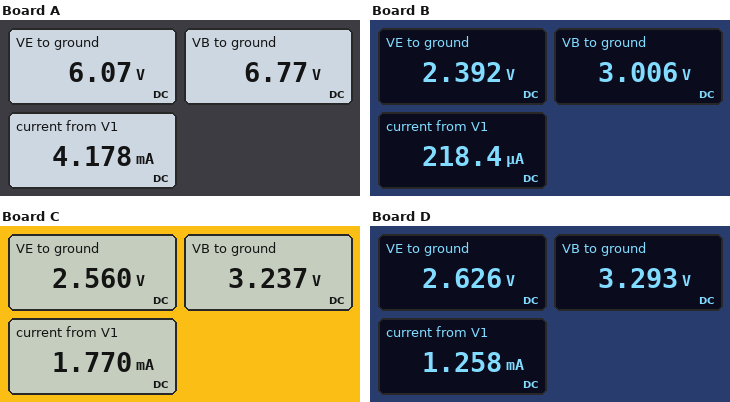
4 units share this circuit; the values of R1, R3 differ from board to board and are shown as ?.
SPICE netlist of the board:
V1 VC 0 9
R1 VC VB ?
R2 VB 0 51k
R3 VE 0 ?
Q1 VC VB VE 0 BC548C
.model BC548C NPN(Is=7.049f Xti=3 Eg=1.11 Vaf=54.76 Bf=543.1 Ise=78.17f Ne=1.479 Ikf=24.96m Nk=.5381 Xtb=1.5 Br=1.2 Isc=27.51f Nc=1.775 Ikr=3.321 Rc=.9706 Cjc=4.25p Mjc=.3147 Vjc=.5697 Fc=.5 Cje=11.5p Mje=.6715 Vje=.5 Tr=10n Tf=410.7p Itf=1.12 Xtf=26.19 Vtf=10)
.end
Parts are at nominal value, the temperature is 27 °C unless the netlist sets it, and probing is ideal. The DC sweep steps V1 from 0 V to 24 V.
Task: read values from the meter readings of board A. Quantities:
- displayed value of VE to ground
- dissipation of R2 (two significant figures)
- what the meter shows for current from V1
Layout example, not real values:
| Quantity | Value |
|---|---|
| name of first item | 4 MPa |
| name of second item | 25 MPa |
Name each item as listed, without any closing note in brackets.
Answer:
| Quantity | Value |
|---|---|
| displayed value of VE to ground | 6.07 V |
| dissipation of R2 | 900 µW |
| what the meter shows for current from V1 | 4.178 mA |
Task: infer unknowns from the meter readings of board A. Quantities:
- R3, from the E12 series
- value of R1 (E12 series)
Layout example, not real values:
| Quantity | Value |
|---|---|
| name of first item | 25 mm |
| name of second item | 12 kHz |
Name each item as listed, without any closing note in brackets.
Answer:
| Quantity | Value |
|---|---|
| R3, from the E12 series | 1.5 kΩ |
| value of R1 | 15 kΩ |
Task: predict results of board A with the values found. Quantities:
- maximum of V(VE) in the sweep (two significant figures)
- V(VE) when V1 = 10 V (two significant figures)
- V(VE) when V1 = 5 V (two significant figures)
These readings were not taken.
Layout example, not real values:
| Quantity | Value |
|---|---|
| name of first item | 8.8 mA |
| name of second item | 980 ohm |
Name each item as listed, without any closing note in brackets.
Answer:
| Quantity | Value |
|---|---|
| maximum of V(VE) in the sweep | 17 V |
| V(VE) when V1 = 10 V | 6.8 V |
| V(VE) when V1 = 5 V | 3.1 V |
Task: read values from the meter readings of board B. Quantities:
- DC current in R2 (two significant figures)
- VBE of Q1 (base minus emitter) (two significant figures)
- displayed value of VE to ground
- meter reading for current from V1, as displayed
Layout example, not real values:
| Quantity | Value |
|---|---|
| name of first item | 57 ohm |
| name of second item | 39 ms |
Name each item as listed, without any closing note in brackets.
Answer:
| Quantity | Value |
|---|---|
| DC current in R2 | 59 µA |
| VBE of Q1 (base minus emitter) | 610 mV |
| displayed value of VE to ground | 2.392 V |
| meter reading for current from V1, as displayed | 218.4 µA |
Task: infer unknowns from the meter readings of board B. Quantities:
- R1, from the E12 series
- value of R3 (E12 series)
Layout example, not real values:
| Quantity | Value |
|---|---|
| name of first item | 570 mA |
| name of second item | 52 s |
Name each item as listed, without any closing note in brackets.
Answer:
| Quantity | Value |
|---|---|
| R1, from the E12 series | 100 kΩ |
| value of R3 | 15 kΩ |
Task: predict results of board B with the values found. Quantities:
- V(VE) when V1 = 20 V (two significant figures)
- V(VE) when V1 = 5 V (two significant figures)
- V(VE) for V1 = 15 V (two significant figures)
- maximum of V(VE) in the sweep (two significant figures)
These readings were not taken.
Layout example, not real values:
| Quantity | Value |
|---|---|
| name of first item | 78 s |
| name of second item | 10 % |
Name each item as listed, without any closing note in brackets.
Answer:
| Quantity | Value |
|---|---|
| V(VE) when V1 = 20 V | 6.1 V |
| V(VE) when V1 = 5 V | 1.1 V |
| V(VE) for V1 = 15 V | 4.4 V |
| maximum of V(VE) in the sweep | 7.4 V |
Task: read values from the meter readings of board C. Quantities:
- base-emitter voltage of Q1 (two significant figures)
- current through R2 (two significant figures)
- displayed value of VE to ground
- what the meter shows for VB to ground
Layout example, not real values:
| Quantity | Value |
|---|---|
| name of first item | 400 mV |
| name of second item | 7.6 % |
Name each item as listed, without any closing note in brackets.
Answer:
| Quantity | Value |
|---|---|
| base-emitter voltage of Q1 | 680 mV |
| current through R2 | 63 µA |
| displayed value of VE to ground | 2.560 V |
| what the meter shows for VB to ground | 3.237 V |
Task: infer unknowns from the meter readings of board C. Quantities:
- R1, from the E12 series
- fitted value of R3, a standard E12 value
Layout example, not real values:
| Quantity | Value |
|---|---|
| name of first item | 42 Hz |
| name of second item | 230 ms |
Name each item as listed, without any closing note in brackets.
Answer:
| Quantity | Value |
|---|---|
| R1, from the E12 series | 82 kΩ |
| fitted value of R3, a standard E12 value | 1.5 kΩ |
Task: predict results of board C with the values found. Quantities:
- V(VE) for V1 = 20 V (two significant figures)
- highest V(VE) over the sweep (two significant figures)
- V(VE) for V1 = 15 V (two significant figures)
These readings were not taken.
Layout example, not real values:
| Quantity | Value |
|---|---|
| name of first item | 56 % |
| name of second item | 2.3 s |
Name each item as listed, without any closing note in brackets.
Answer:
| Quantity | Value |
|---|---|
| V(VE) for V1 = 20 V | 6.5 V |
| highest V(VE) over the sweep | 8.0 V |
| V(VE) for V1 = 15 V | 4.7 V |
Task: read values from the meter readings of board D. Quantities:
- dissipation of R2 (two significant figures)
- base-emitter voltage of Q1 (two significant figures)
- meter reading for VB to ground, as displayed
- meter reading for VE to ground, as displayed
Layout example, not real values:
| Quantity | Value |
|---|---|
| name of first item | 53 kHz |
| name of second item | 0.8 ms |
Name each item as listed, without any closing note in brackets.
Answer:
| Quantity | Value |
|---|---|
| dissipation of R2 | 210 µW |
| base-emitter voltage of Q1 | 670 mV |
| meter reading for VB to ground, as displayed | 3.293 V |
| meter reading for VE to ground, as displayed | 2.626 V |
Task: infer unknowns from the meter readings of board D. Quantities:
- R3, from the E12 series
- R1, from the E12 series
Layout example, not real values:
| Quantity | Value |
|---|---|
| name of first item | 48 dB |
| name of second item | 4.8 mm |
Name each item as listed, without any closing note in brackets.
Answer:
| Quantity | Value |
|---|---|
| R3, from the E12 series | 2.2 kΩ |
| R1, from the E12 series | 82 kΩ |
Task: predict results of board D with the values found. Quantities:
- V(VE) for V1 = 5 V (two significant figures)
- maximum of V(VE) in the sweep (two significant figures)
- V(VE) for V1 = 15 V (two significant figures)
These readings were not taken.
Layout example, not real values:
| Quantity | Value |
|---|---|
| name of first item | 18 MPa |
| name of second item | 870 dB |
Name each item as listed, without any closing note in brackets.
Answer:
| Quantity | Value |
|---|---|
| V(VE) for V1 = 5 V | 1.2 V |
| maximum of V(VE) in the sweep | 8.1 V |
| V(VE) for V1 = 15 V | 4.8 V |
